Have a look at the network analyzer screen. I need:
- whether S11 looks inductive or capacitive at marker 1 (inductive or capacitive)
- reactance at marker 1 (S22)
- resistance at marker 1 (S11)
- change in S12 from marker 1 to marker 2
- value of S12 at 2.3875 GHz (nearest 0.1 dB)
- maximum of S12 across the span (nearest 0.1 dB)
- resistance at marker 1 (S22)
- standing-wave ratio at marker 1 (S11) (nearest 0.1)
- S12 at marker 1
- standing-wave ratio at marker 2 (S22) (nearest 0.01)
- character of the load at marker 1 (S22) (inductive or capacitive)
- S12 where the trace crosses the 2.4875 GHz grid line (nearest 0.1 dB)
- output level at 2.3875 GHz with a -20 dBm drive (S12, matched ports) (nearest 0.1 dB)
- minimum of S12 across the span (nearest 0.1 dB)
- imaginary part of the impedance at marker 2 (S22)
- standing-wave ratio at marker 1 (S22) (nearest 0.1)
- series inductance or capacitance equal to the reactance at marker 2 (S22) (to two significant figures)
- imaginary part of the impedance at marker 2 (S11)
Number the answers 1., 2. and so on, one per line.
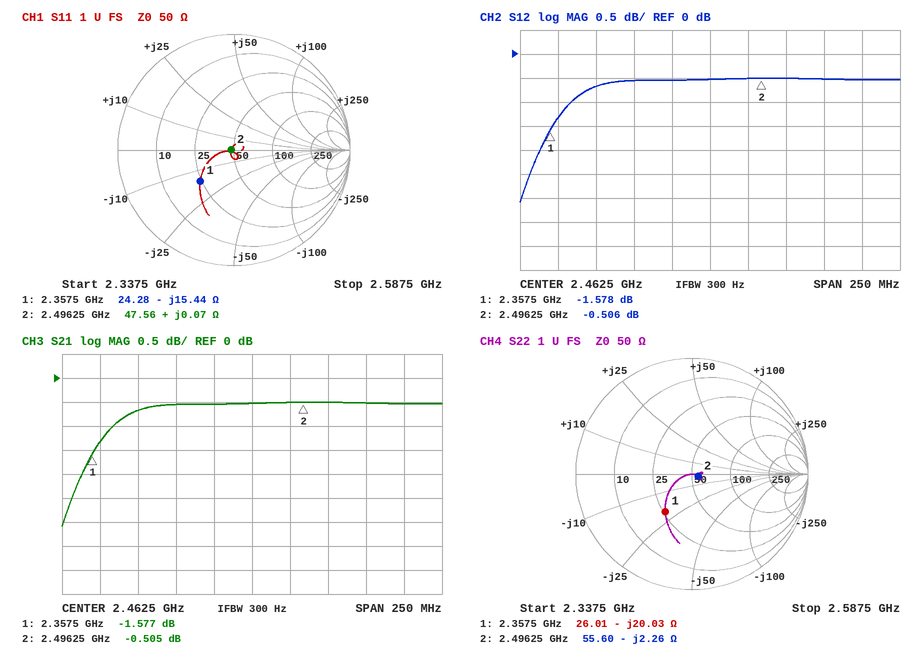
1. capacitive
2. -20.03 Ω
3. 24.28 Ω
4. 1.072 dB
5. -0.7 dB
6. -0.5 dB
7. 26.01 Ω
8. 2.3
9. -1.578 dB
10. 1.12
11. capacitive
12. -0.5 dB
13. -20.7 dBm
14. -3.1 dB
15. -2.26 Ω
16. 2.3
17. 28 pF
18. +0.07 Ω
